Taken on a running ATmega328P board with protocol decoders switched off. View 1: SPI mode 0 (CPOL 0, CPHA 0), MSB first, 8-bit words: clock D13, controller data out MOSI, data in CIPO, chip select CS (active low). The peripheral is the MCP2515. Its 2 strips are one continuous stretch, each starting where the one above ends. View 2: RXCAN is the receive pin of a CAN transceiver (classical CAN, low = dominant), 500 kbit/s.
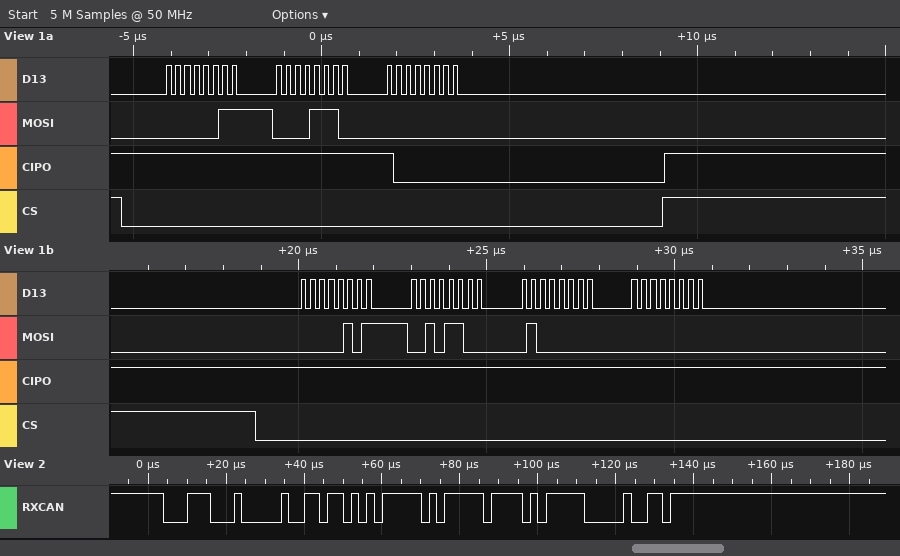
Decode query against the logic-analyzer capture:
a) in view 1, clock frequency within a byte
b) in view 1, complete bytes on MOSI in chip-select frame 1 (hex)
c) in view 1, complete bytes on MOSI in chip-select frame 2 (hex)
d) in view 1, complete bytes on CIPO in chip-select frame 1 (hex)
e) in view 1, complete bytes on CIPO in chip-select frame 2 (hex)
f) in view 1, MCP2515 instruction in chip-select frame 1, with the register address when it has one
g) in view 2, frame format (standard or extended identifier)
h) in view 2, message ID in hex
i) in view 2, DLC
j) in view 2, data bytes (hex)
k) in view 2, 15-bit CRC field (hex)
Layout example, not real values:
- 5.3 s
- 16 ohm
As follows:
- 4 MHz
- 03 0E 00
- 05 2C 40 00
- FF FF 80
- FF FF FF FF
- READ 0x0E
- standard
- 0x1C4
- 3
- 6A FD FF
- 0x2F81
